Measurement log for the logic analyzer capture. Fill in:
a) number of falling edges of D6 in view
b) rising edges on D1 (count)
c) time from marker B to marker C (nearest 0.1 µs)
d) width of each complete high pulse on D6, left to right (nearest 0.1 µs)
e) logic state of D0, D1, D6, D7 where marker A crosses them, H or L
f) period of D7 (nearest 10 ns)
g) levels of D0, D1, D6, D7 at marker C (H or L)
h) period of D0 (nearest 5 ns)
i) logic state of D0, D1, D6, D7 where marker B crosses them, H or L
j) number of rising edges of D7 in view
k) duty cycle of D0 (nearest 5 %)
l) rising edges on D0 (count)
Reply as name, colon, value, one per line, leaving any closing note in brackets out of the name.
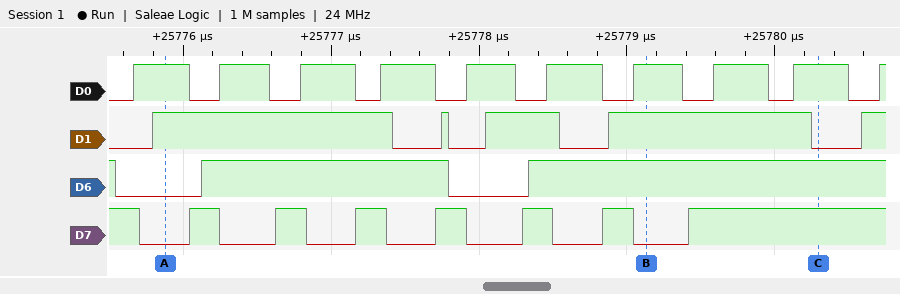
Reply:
number of falling edges of D6 in view: 2
rising edges on D1: 5
time from marker B to marker C: 1.2 µs
width of each complete high pulse on D6, left to right: 1.7 µs
logic state of D0, D1, D6, D7 where marker A crosses them, H or L: D0=H, D1=H, D6=L, D7=L
period of D7: 560 ns
levels of D0, D1, D6, D7 at marker C: D0=H, D1=L, D6=H, D7=H
period of D0: 560 ns
logic state of D0, D1, D6, D7 where marker B crosses them, H or L: D0=H, D1=H, D6=H, D7=L
number of rising edges of D7 in view: 7
duty cycle of D0: 65 %
rising edges on D0: 10
